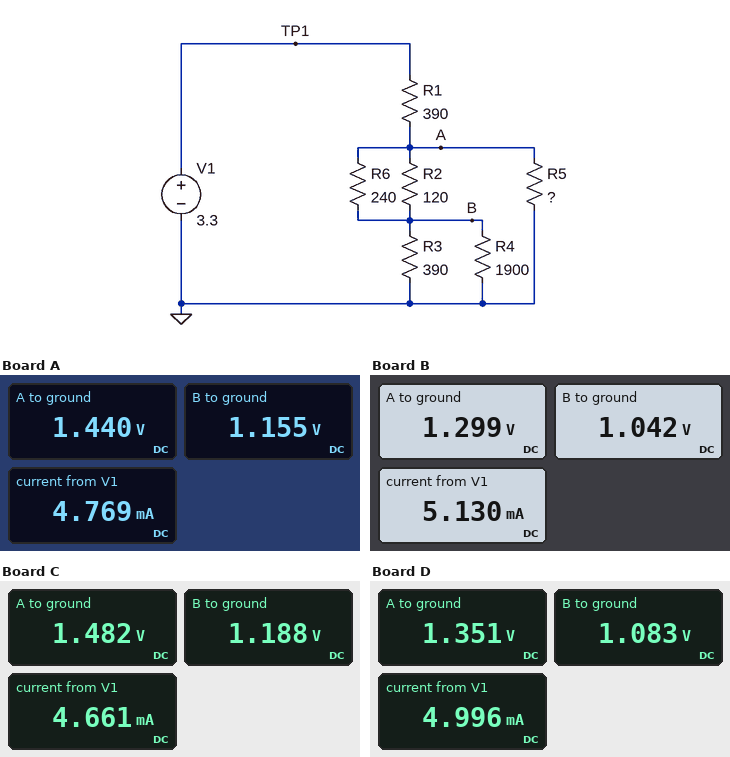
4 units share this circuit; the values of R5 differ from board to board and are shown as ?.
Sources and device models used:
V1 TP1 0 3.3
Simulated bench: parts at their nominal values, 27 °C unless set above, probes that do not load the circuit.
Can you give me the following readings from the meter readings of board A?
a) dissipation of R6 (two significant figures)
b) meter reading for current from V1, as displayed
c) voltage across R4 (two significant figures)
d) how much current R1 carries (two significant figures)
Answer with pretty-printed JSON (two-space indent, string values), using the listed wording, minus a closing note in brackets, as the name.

{
  "dissipation of R6": "340 µW",
  "meter reading for current from V1, as displayed": "4.769 mA",
  "voltage across R4": "1.2 V",
  "how much current R1 carries": "4.8 mA"
}
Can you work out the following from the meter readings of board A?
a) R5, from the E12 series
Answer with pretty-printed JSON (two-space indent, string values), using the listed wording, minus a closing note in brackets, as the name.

{
  "R5, from the E12 series": "1.2 kΩ"
}
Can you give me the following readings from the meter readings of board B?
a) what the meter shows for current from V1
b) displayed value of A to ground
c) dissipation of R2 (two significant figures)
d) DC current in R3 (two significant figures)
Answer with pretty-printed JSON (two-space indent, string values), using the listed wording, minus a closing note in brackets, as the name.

{
  "what the meter shows for current from V1": "5.130 mA",
  "displayed value of A to ground": "1.299 V",
  "dissipation of R2": "550 µW",
  "DC current in R3": "2.7 mA"
}
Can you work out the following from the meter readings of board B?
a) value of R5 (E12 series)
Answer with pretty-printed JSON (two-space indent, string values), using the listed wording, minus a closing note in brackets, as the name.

{
  "value of R5": "680 Ω"
}
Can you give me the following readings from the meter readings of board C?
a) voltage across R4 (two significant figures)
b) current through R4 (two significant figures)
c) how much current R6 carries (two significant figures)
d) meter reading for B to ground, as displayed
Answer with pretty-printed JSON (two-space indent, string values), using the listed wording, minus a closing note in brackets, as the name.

{
  "voltage across R4": "1.2 V",
  "current through R4": "630 µA",
  "how much current R6 carries": "1.2 mA",
  "meter reading for B to ground, as displayed": "1.188 V"
}
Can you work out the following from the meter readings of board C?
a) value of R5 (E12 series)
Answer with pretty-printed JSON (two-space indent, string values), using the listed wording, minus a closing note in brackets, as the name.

{
  "value of R5": "1.5 kΩ"
}
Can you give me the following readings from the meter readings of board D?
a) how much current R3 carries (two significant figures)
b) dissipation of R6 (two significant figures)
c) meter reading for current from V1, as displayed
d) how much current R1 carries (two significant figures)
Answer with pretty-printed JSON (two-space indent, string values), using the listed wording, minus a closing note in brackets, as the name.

{
  "how much current R3 carries": "2.8 mA",
  "dissipation of R6": "300 µW",
  "meter reading for current from V1, as displayed": "4.996 mA",
  "how much current R1 carries": "5.0 mA"
}
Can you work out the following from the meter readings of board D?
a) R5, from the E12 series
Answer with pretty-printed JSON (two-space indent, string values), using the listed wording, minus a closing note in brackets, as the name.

{
  "R5, from the E12 series": "820 Ω"
}
